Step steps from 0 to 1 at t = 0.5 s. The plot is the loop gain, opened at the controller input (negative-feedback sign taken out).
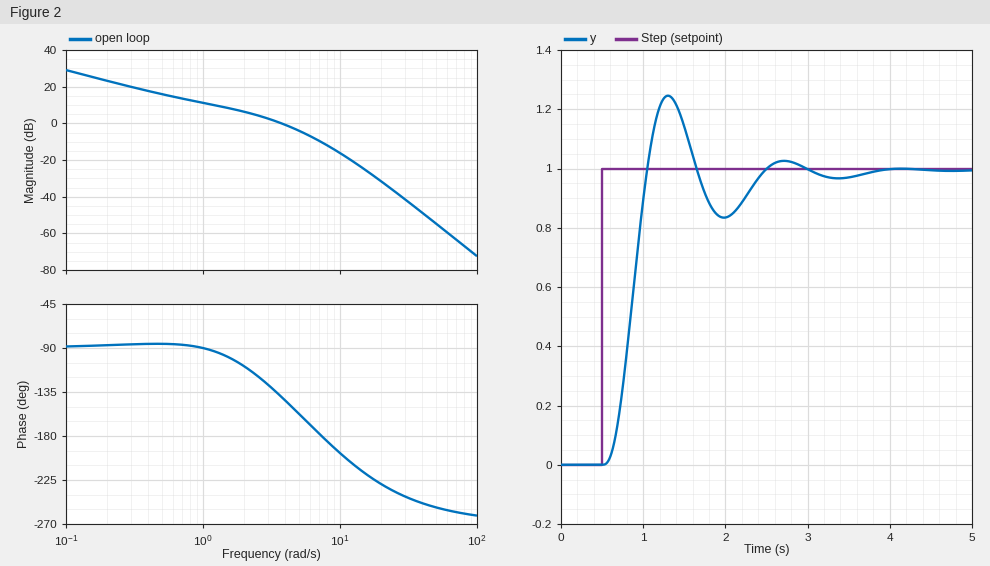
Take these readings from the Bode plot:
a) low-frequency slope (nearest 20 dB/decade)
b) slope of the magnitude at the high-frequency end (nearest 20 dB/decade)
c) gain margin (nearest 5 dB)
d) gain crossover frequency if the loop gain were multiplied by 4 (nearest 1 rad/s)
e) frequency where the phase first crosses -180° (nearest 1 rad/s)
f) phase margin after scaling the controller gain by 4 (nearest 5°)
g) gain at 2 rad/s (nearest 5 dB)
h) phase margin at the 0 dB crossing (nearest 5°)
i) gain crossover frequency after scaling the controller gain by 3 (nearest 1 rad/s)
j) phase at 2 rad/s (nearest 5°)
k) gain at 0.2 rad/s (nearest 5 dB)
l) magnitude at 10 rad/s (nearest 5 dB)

-20 dB/decade
-60 dB/decade
10 dB
8 rad/s
7 rad/s
-5°
5 dB
40°
7 rad/s
-110°
25 dB
-15 dB
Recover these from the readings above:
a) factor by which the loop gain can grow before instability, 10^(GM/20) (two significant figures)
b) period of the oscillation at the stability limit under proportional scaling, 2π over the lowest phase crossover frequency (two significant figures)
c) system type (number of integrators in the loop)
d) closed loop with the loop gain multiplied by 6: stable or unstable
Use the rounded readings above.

3.2
0.90 s
1
unstable
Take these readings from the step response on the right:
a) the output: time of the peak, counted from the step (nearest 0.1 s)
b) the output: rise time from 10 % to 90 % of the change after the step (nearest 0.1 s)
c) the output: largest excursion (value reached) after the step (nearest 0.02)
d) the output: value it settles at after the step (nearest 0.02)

0.8 s
0.3 s
1.24
1.00
